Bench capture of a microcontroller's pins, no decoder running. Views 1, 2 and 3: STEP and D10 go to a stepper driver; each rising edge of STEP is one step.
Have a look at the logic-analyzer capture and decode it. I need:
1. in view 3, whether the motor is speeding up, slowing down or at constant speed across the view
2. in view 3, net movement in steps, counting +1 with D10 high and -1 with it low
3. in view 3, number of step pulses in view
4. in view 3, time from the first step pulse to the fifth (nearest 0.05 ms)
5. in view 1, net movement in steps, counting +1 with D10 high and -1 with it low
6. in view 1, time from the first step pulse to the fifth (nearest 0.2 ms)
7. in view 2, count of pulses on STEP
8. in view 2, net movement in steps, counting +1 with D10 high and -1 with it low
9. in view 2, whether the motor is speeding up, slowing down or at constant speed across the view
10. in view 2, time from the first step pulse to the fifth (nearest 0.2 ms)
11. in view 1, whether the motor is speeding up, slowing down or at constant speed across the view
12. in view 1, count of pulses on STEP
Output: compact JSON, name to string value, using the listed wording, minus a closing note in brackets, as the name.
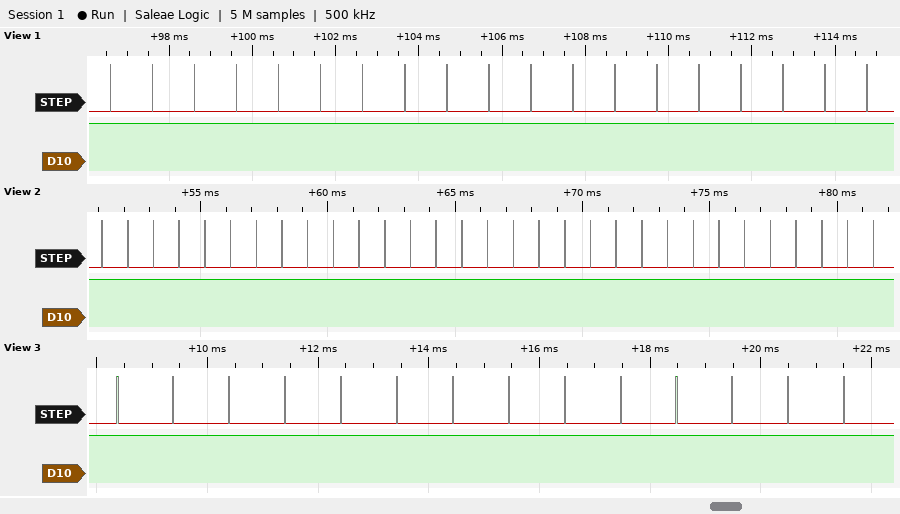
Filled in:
{"in view 3, whether the motor is speeding up, slowing down or at constant speed across the view": "constant speed", "in view 3, net movement in steps, counting +1 with D10 high and -1 with it low": "+14", "in view 3, number of step pulses in view": "14", "in view 3, time from the first step pulse to the fifth": "4.05 ms", "in view 1, net movement in steps, counting +1 with D10 high and -1 with it low": "+19", "in view 1, time from the first step pulse to the fifth": "4.0 ms", "in view 2, count of pulses on STEP": "31", "in view 2, net movement in steps, counting +1 with D10 high and -1 with it low": "+31", "in view 2, whether the motor is speeding up, slowing down or at constant speed across the view": "constant speed", "in view 2, time from the first step pulse to the fifth": "4.0 ms", "in view 1, whether the motor is speeding up, slowing down or at constant speed across the view": "constant speed", "in view 1, count of pulses on STEP": "19"}
